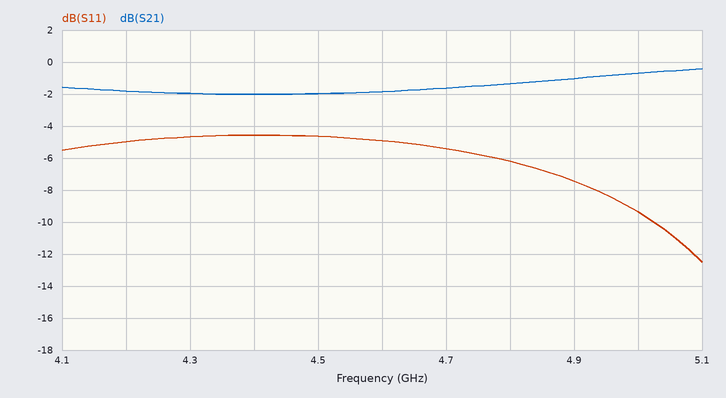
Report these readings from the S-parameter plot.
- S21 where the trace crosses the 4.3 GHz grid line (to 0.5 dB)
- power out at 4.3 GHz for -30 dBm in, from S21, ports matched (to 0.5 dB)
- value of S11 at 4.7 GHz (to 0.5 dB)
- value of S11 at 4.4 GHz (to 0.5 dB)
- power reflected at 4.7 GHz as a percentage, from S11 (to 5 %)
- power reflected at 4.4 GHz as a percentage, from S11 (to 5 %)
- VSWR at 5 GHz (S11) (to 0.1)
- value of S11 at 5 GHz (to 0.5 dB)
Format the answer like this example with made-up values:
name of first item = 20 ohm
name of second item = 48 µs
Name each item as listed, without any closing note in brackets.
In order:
S21 where the trace crosses the 4.3 GHz grid line = -2.0 dB
power out at 4.3 GHz for -30 dBm in, from S21, ports matched = -32.0 dBm
value of S11 at 4.7 GHz = -5.5 dB
value of S11 at 4.4 GHz = -4.5 dB
power reflected at 4.7 GHz as a percentage, from S11 = 30 %
power reflected at 4.4 GHz as a percentage, from S11 = 35 %
VSWR at 5 GHz (S11) = 2.0
value of S11 at 5 GHz = -9.5 dB
